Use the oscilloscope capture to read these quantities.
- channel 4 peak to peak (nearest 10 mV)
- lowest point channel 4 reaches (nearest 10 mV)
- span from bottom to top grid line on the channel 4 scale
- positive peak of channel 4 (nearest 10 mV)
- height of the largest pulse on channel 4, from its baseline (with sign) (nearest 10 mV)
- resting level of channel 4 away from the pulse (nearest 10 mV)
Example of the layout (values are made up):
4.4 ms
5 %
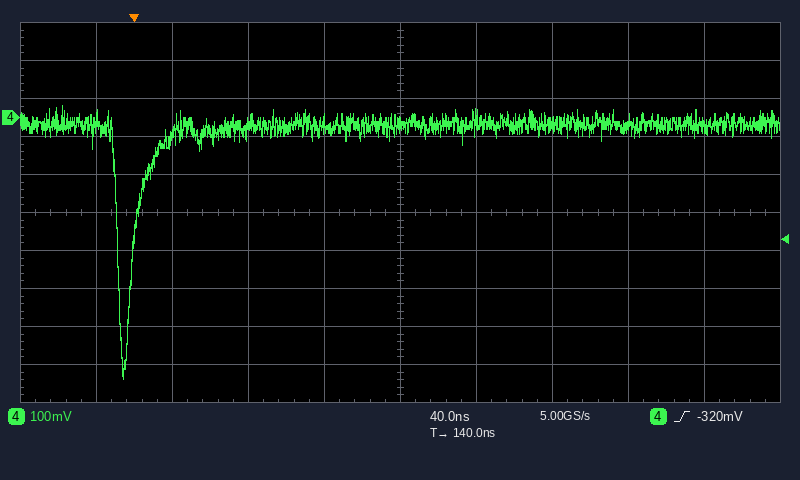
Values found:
720 mV
-690 mV
1 V
30 mV
-670 mV
-20 mV
